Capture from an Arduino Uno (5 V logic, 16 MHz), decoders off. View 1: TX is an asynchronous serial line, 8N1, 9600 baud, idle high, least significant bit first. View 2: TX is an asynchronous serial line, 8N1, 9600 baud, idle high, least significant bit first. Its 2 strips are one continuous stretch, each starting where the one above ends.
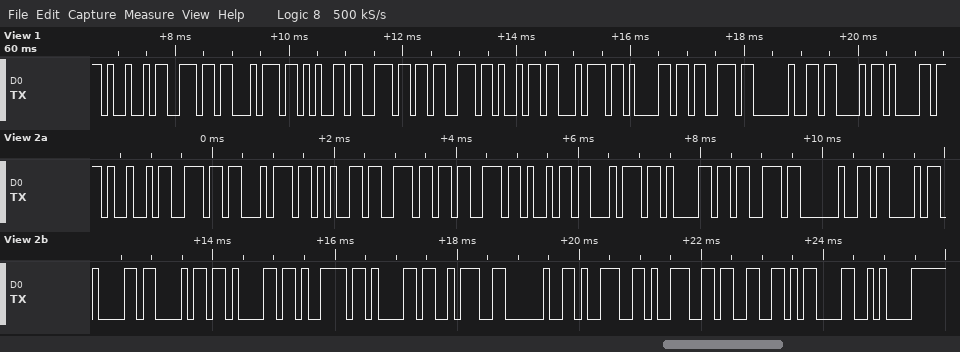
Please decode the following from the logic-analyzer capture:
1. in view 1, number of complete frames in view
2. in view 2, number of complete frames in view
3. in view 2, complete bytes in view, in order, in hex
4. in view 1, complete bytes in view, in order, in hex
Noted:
13
24
0x49 0x6E 0x74 0x65 0x6E 0x73 0x69 0x74 0x61 0x73 0x20 0x43 0x61 0x68 0x61 0x79 0x61 0x3A 0x20 0x39 0x39 0x33 0x0D 0x0A
49 6E 74 65 6E 73 69 74 61 73 20 43 61
